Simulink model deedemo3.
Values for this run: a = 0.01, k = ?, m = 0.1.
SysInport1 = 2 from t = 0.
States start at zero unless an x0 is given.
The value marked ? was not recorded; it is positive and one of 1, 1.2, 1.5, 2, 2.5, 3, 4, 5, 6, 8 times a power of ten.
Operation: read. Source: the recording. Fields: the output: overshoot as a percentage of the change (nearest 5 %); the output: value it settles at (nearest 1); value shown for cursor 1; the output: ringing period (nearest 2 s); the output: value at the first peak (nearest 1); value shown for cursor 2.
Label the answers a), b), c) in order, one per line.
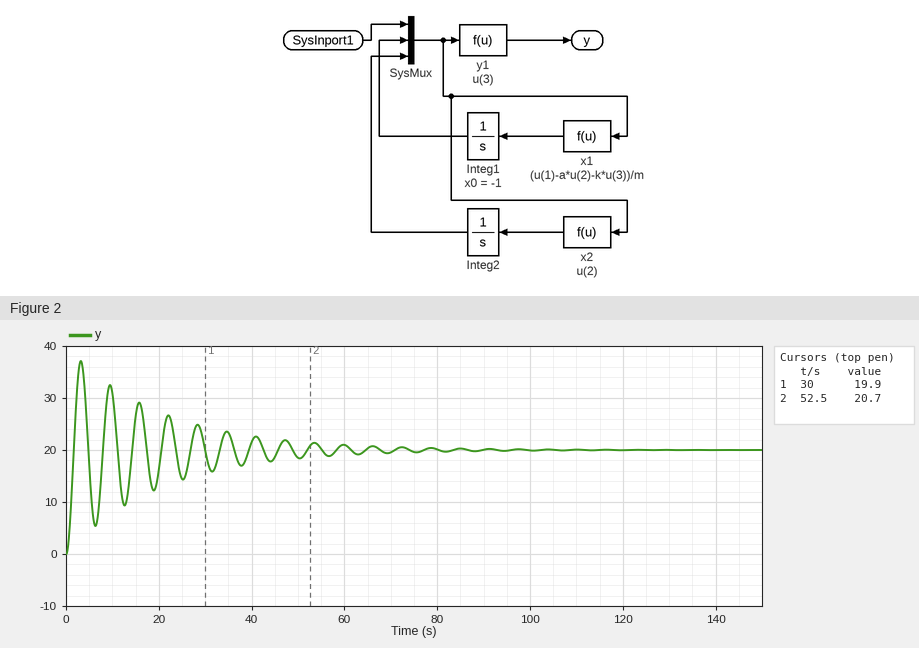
a) 85 %
b) 20
c) 19.9
d) 6 s
e) 37
f) 20.7
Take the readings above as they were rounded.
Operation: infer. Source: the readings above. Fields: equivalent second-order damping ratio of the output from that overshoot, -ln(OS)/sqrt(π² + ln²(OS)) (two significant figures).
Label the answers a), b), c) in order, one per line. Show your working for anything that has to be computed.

a) ln(0.85) = -0.163; 0.163 / sqrt(9.870 + 0.026) = 0.052
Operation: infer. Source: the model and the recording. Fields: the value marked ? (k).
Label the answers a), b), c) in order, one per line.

a) 0.1
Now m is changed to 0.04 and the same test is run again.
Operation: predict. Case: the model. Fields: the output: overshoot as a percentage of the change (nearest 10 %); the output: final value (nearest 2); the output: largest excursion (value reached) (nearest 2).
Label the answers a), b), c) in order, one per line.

a) 80 %
b) 20
c) 36
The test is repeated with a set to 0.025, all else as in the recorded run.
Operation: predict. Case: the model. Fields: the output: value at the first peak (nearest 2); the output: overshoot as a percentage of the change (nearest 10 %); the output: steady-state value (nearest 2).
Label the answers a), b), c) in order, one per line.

a) 34
b) 70 %
c) 20
